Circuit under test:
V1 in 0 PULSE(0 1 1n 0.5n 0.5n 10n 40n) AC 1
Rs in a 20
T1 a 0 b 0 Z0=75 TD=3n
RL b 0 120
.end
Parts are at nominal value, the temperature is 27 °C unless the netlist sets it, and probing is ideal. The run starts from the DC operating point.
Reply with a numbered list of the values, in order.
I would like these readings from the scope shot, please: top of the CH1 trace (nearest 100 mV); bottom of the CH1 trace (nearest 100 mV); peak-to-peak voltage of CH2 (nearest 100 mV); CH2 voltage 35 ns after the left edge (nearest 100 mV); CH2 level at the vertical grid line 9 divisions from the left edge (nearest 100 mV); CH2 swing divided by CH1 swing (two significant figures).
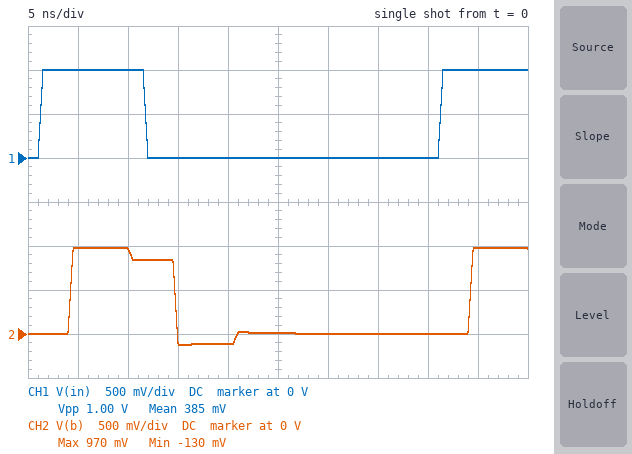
1. 1.0 V
2. 0 V
3. 1.1 V
4. 0 V
5. 1.0 V
6. 1.1
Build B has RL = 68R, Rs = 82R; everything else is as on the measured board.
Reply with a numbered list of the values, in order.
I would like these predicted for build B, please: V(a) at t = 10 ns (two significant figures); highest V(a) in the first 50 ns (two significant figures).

1. 450 mV
2. 480 mV
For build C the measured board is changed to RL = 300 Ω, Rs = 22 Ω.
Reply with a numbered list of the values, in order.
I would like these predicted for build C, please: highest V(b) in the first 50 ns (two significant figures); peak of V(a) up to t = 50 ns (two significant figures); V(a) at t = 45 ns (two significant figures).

1. 1.2 V
2. 980 mV
3. 770 mV
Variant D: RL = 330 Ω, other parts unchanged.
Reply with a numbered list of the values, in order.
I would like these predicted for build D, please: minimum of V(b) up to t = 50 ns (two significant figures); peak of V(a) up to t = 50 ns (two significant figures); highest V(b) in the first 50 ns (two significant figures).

1. -470 mV
2. 1.0 V
3. 1.3 V
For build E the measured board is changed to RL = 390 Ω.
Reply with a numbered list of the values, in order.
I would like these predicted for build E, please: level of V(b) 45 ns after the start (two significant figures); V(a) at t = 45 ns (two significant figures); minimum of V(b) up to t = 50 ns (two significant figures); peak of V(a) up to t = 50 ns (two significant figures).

1. 1.3 V
2. 790 mV
3. -520 mV
4. 1.0 V
